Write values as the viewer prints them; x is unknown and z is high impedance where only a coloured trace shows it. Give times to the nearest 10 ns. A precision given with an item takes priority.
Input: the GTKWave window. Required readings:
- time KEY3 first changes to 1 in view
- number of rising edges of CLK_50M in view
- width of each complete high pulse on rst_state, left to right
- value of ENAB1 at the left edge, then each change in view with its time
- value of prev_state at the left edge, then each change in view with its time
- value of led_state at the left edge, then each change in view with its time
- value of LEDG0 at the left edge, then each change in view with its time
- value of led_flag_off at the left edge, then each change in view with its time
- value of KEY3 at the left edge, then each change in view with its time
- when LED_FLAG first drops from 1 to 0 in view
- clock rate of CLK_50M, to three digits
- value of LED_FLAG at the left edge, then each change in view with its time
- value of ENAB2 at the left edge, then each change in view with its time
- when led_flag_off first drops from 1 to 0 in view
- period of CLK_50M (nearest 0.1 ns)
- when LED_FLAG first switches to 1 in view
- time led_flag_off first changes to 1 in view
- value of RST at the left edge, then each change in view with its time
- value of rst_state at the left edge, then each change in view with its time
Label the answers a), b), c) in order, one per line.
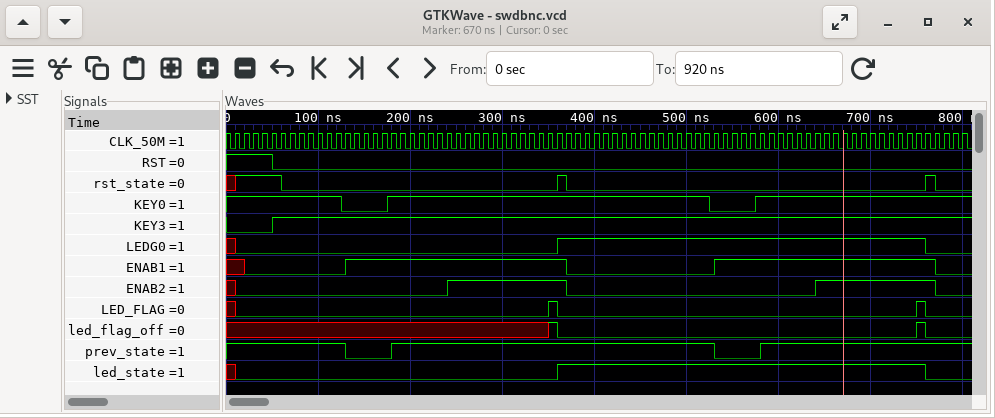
a) 50 ns
b) 80
c) 10 ns, 10 ns
d) x, 0 at 20 ns, 1 at 130 ns, 0 at 370 ns, 1 at 530 ns, 0 at 770 ns
e) 1, 0 at 130 ns, 1 at 180 ns, 0 at 530 ns, 1 at 580 ns
f) x, 0 at 10 ns, 1 at 360 ns, 0 at 760 ns
g) x, 0 at 10 ns, 1 at 360 ns, 0 at 760 ns
h) x, 1 at 350 ns, 0 at 360 ns, 1 at 750 ns, 0 at 760 ns
i) 0, 1 at 50 ns
j) 360 ns
k) 100 MHz
l) x, 0 at 10 ns, 1 at 350 ns, 0 at 360 ns, 1 at 750 ns, 0 at 760 ns
m) x, 0 at 10 ns, 1 at 240 ns, 0 at 370 ns, 1 at 640 ns, 0 at 770 ns
n) 360 ns
o) 10 ns
p) 350 ns
q) 350 ns
r) 1, 0 at 50 ns
s) x, 1 at 10 ns, 0 at 60 ns, 1 at 360 ns, 0 at 370 ns, 1 at 760 ns, 0 at 770 ns
